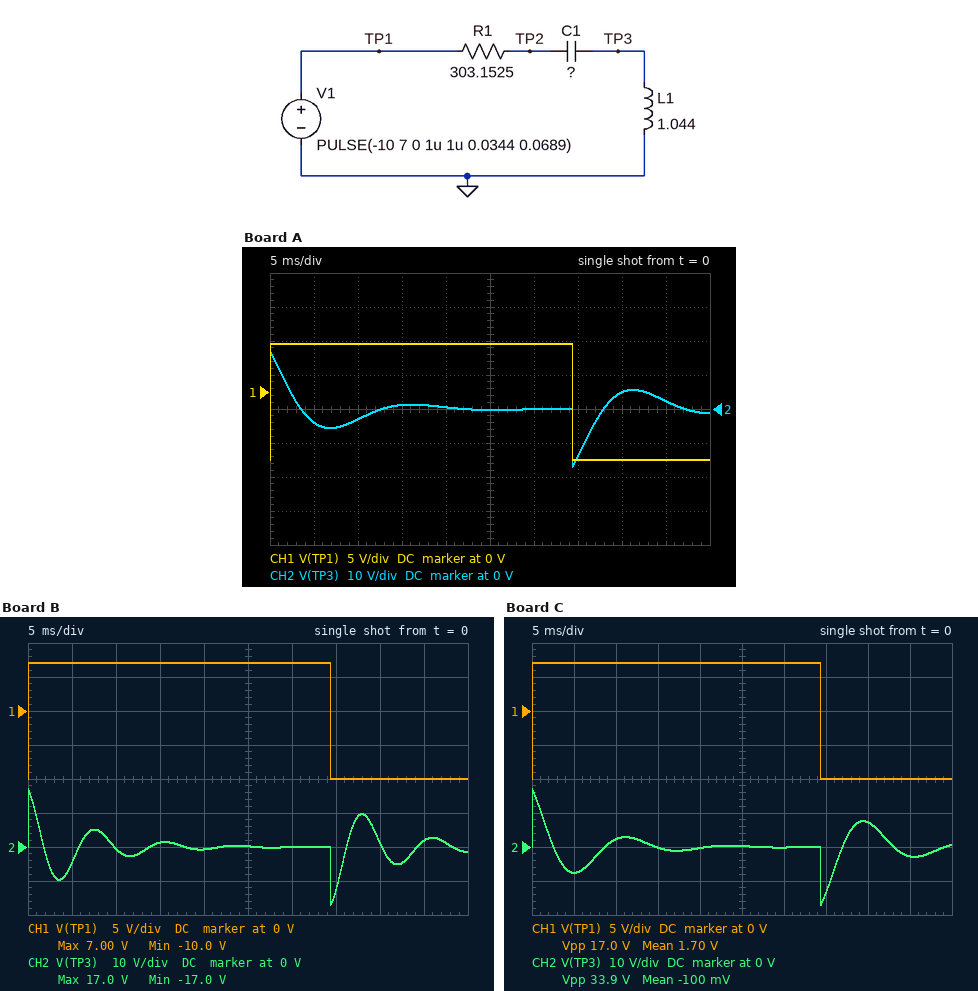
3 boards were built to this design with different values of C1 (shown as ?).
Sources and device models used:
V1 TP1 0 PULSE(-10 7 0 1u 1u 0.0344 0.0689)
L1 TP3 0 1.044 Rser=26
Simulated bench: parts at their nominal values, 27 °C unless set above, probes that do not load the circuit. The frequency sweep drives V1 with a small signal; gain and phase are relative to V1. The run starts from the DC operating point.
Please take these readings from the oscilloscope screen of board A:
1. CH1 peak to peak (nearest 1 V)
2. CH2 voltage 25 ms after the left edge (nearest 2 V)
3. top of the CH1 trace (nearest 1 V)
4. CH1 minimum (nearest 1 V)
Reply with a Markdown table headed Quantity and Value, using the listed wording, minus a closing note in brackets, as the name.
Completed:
| Quantity | Value |
|---|---|
| CH1 peak to peak | 17 V |
| CH2 voltage 25 ms after the left edge | 0 V |
| top of the CH1 trace | 7 V |
| CH1 minimum | -10 V |
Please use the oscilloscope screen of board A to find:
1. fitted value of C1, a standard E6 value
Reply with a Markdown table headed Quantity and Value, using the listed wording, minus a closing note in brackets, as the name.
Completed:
| Quantity | Value |
|---|---|
| fitted value of C1, a standard E6 value | 6.8 µF |
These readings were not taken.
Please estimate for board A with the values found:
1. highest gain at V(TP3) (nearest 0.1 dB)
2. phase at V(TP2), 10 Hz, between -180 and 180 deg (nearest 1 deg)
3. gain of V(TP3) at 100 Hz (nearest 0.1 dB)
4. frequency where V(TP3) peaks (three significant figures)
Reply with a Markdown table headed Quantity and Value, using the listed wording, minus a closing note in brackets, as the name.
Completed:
| Quantity | Value |
|---|---|
| highest gain at V(TP3) | 2.4 dB |
| phase at V(TP2), 10 Hz, between -180 and 180 deg | -8 deg |
| gain of V(TP3) at 100 Hz | 1.8 dB |
| frequency where V(TP3) peaks | 74.2 Hz |
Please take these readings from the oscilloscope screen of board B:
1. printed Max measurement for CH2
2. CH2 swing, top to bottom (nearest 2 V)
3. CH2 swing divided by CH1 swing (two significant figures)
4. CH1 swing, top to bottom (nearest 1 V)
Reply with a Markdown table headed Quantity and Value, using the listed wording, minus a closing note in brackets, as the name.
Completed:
| Quantity | Value |
|---|---|
| printed Max measurement for CH2 | 17.0 V |
| CH2 swing, top to bottom | 34 V |
| CH2 swing divided by CH1 swing | 2.0 |
| CH1 swing, top to bottom | 17 V |
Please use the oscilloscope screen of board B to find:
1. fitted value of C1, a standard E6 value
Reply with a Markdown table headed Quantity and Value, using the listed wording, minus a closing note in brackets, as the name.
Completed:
| Quantity | Value |
|---|---|
| fitted value of C1, a standard E6 value | 1.5 µF |
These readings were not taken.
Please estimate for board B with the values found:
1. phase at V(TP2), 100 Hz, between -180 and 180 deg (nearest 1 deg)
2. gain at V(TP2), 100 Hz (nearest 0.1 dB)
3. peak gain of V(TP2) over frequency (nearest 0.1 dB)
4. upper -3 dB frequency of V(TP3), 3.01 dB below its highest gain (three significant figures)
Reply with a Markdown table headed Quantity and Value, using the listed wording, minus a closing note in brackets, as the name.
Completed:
| Quantity | Value |
|---|---|
| phase at V(TP2), 100 Hz, between -180 and 180 deg | -35 deg |
| gain at V(TP2), 100 Hz | -2.2 dB |
| peak gain of V(TP2) over frequency | 0 dB |
| upper -3 dB frequency of V(TP3), 3.01 dB below its highest gain | 174 Hz |
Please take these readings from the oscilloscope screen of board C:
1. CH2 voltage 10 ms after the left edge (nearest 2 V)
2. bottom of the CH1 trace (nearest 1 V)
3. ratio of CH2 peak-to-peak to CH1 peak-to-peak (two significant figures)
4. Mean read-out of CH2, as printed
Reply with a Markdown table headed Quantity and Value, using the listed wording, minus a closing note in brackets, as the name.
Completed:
| Quantity | Value |
|---|---|
| CH2 voltage 10 ms after the left edge | 2 V |
| bottom of the CH1 trace | -10 V |
| ratio of CH2 peak-to-peak to CH1 peak-to-peak | 2.0 |
| Mean read-out of CH2, as printed | -100 mV |
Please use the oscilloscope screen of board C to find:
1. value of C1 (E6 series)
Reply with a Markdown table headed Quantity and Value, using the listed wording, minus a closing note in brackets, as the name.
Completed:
| Quantity | Value |
|---|---|
| value of C1 | 3.3 µF |
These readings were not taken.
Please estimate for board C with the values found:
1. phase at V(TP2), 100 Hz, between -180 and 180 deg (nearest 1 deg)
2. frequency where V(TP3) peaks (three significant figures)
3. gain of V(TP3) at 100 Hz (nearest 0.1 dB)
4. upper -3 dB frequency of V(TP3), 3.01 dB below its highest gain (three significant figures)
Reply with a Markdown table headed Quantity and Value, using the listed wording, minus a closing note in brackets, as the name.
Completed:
| Quantity | Value |
|---|---|
| phase at V(TP2), 100 Hz, between -180 and 180 deg | 54 deg |
| frequency where V(TP3) peaks | 94.2 Hz |
| gain of V(TP3) at 100 Hz | 4.9 dB |
| upper -3 dB frequency of V(TP3), 3.01 dB below its highest gain | 165 Hz |
